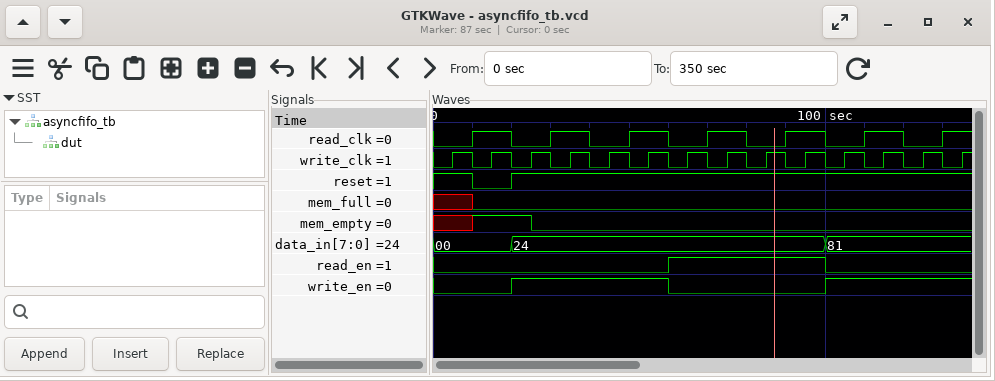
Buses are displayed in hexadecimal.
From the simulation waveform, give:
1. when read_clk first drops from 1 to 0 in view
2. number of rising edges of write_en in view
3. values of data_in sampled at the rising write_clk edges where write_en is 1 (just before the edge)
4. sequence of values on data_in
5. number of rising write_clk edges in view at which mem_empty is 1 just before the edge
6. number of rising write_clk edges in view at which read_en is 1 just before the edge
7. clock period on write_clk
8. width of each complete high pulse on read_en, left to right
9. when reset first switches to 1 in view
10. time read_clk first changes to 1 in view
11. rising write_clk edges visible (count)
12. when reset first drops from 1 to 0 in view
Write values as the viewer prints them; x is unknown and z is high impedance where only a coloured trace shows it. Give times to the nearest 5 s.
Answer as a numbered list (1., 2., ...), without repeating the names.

1. 20 s
2. 2
3. 24, 24, 24, 24, 81, 81, 81, 81
4. 00, 24, 81
5. 2
6. 4
7. 10 s
8. 40 s
9. 20 s
10. 10 s
11. 14
12. 10 s
